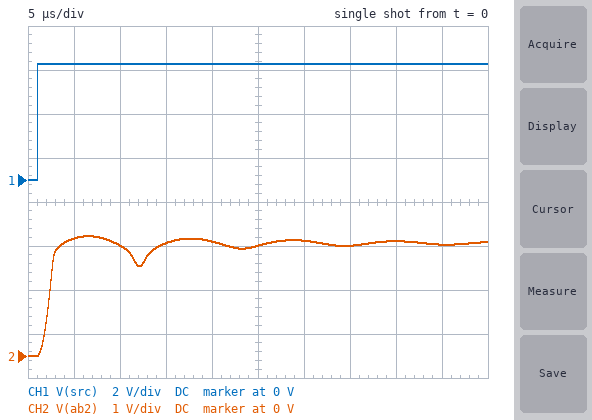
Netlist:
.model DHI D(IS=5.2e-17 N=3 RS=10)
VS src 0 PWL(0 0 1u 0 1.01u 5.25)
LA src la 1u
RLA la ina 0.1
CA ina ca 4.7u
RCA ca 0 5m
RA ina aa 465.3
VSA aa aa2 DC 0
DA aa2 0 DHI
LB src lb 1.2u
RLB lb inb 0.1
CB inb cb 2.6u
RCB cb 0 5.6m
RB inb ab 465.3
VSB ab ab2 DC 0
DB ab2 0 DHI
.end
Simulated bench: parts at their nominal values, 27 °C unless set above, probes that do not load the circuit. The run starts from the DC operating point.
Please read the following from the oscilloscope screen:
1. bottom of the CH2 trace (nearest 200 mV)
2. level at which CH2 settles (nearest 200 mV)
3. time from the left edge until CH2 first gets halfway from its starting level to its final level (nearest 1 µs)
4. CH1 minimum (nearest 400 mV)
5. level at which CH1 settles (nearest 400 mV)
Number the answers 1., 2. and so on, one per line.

1. 0 V
2. 2.6 V
3. 2 µs
4. 0 V
5. 5.2 V
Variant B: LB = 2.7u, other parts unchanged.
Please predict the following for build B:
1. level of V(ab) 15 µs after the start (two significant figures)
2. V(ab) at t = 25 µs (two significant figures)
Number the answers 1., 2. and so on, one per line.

1. 2.4 V
2. 2.7 V
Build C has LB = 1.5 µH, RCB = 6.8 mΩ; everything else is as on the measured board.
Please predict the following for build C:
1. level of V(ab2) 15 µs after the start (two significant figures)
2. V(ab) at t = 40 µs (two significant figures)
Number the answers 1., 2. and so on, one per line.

1. 2.4 V
2. 2.5 V
